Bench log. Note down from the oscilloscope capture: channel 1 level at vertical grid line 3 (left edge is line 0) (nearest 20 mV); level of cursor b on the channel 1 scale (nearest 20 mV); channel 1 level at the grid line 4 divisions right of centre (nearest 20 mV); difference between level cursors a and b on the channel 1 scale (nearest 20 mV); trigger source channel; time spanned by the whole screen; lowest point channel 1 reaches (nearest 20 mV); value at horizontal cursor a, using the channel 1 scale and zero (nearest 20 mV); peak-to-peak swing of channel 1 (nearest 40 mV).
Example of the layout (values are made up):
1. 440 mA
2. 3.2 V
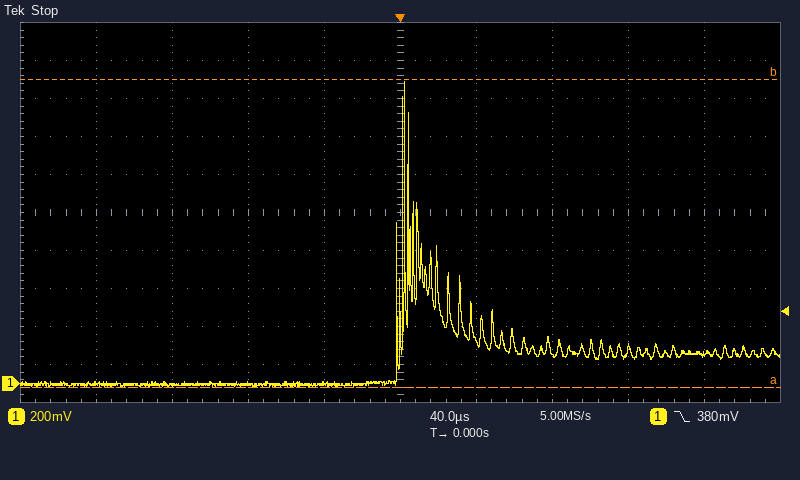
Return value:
1. 0 mV
2. 1.60 V
3. 160 mV
4. 1.62 V
5. channel 1
6. 400 µs
7. -20 mV
8. -20 mV
9. 1.60 V
